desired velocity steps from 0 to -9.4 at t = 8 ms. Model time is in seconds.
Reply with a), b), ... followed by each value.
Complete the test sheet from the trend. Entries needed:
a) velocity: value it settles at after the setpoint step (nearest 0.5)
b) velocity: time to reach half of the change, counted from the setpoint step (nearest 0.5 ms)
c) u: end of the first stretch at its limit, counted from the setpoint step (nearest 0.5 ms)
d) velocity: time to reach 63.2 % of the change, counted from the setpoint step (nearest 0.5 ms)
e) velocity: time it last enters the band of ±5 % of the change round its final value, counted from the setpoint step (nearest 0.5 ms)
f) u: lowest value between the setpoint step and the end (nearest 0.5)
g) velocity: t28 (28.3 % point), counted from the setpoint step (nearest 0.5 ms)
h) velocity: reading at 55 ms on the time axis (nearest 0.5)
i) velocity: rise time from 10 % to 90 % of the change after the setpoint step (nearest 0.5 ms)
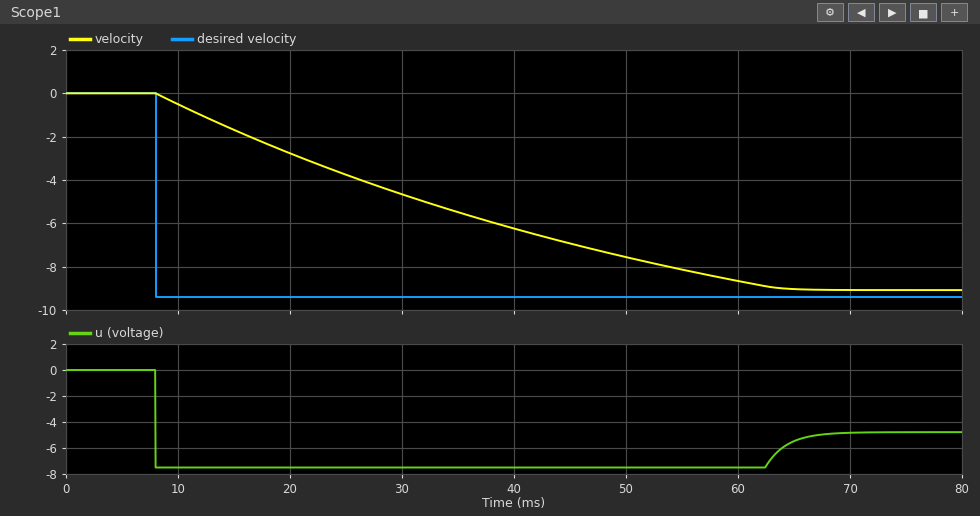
a) -9.0
b) 21.5 ms
c) 54.5 ms
d) 28.5 ms
e) 51.5 ms
f) -7.5
g) 11.0 ms
h) -8.0
i) 43.5 ms
